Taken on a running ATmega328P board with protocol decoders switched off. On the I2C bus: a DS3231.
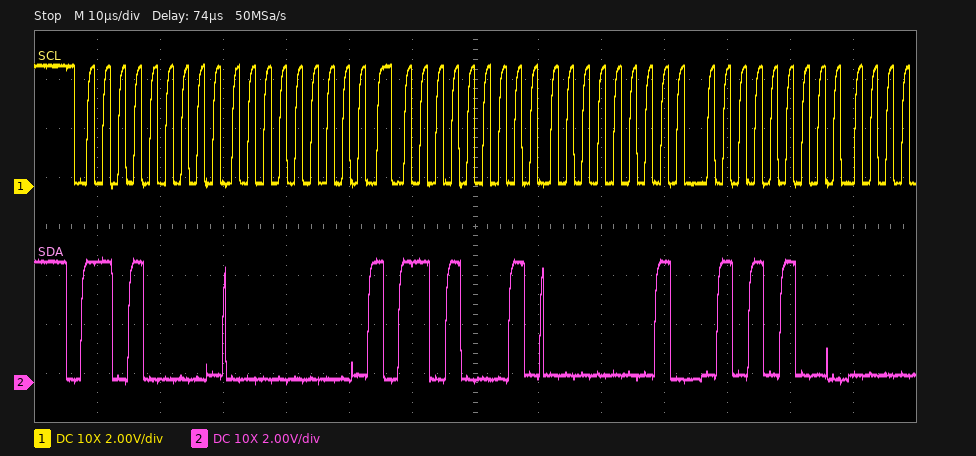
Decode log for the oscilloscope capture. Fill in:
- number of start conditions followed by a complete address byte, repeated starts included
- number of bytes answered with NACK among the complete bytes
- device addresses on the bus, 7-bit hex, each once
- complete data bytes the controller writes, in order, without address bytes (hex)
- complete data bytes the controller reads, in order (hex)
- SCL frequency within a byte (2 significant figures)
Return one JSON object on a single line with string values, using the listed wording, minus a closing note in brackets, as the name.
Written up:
{"number of start conditions followed by a complete address byte, repeated starts included": "2", "number of bytes answered with NACK among the complete bytes": "0", "device addresses on the bus, 7-bit hex, each once": "0x68", "complete data bytes the controller writes, in order, without address bytes": "00", "complete data bytes the controller reads, in order": "01 54", "SCL frequency within a byte": "400 kHz"}
